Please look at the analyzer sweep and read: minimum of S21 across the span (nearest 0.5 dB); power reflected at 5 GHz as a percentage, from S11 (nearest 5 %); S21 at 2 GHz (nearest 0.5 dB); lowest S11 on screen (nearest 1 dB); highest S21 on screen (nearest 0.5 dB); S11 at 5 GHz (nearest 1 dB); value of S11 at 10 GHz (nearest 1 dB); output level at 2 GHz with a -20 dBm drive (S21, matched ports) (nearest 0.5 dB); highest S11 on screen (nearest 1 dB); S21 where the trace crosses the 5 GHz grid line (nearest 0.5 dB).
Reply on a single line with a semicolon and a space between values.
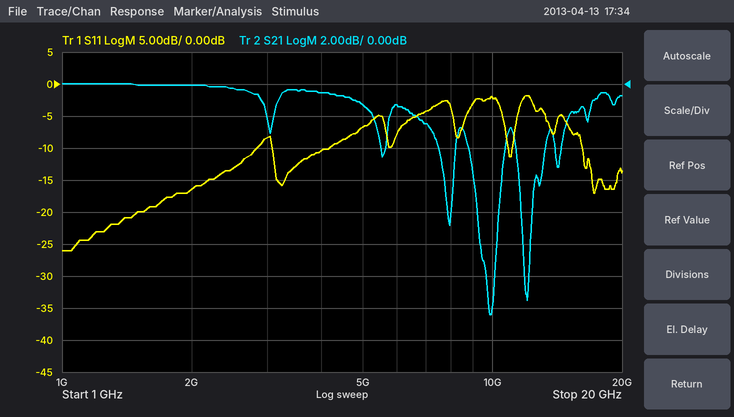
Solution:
-14.5 dB; 20 %; 0.0 dB; -26 dB; 0.0 dB; -7 dB; -2 dB; -20.0 dBm; -2 dB; -1.5 dB
